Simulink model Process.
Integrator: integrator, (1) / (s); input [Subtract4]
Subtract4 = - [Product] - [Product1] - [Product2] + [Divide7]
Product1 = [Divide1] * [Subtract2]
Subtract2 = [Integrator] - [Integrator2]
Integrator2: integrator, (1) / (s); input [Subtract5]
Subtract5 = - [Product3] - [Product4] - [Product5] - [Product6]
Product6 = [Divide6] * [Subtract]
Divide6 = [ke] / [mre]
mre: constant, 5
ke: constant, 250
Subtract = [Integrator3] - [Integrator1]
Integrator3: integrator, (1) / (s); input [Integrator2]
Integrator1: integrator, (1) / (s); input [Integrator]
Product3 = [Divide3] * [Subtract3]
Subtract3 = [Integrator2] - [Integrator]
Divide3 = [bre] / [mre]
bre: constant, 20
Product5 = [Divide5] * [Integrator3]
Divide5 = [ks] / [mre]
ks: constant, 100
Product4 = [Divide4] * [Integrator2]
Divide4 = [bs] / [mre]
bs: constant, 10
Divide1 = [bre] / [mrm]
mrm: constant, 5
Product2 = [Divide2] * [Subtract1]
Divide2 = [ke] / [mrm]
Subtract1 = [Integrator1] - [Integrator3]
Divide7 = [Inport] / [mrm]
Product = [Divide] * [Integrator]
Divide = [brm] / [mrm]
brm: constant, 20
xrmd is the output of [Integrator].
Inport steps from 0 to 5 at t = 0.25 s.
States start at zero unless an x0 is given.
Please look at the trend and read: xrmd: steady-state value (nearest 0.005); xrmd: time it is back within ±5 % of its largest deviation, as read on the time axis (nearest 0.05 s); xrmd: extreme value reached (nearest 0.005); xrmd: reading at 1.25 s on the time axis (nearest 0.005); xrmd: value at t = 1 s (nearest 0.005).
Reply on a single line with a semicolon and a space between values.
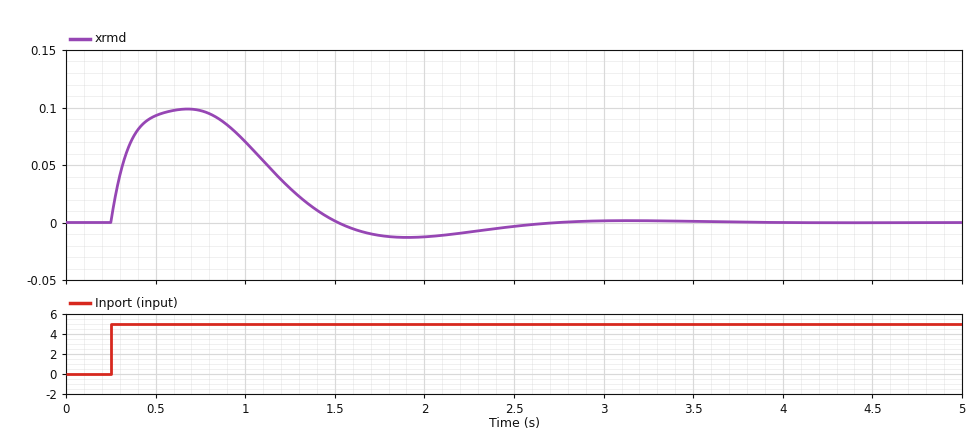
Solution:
0.000; 2.40 s; 0.100; 0.030; 0.070
